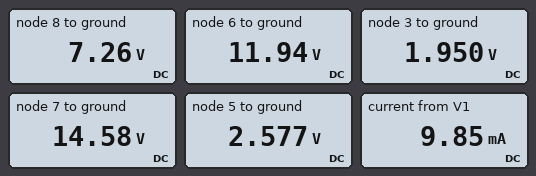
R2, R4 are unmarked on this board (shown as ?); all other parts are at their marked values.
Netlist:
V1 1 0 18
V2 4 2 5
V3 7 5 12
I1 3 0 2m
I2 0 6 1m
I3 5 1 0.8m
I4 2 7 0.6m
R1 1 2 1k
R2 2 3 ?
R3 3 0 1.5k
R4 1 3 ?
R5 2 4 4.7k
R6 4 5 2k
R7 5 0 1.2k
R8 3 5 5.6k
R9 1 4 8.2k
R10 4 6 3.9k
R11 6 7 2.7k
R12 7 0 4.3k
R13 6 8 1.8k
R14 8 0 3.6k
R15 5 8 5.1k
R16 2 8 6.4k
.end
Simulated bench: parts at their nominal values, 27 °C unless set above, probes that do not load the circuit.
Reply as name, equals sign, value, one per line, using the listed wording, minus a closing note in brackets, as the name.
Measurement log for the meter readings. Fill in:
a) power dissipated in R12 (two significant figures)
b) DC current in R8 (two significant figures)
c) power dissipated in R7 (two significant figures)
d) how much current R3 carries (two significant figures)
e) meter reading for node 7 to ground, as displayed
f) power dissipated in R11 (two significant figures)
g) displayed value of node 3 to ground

power dissipated in R12 = 49 mW
DC current in R8 = 110 µA
power dissipated in R7 = 5.5 mW
how much current R3 carries = 1.3 mA
meter reading for node 7 to ground, as displayed = 14.58 V
power dissipated in R11 = 2.6 mW
displayed value of node 3 to ground = 1.950 V
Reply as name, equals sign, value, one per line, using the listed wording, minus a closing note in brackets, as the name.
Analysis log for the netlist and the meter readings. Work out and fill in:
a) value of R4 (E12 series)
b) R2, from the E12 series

value of R4 = 10 kΩ
R2, from the E12 series = 4.7 kΩ
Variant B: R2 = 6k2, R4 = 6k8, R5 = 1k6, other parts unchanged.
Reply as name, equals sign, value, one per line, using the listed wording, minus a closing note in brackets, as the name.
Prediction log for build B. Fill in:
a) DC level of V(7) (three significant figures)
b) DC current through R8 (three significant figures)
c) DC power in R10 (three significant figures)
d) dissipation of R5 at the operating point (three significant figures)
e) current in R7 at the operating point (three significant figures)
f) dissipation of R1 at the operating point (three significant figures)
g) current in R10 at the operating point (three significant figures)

DC level of V(7) = 14.7 V
DC current through R8 = 66.0 µA
DC power in R10 = 1.67 mW
dissipation of R5 at the operating point = 15.6 mW
current in R7 at the operating point = 2.25 mA
dissipation of R1 at the operating point = 69.8 mW
current in R10 at the operating point = 654 µA
